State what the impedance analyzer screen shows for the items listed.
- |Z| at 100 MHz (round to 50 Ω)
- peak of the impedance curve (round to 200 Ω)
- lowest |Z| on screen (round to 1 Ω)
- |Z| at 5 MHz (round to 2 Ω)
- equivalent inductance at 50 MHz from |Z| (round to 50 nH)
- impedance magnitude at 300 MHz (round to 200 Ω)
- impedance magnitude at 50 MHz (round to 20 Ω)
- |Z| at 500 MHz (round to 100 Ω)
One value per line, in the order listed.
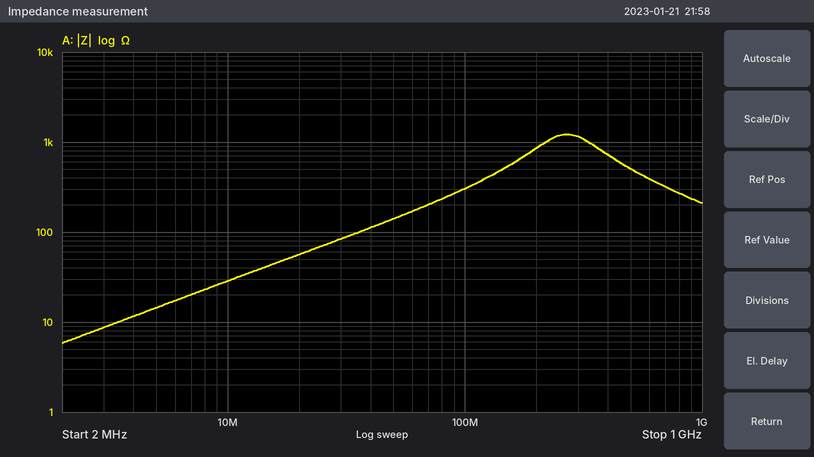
300 Ω
1.2 kΩ
6 Ω
14 Ω
450 nH
1.2 kΩ
140 Ω
500 Ω
